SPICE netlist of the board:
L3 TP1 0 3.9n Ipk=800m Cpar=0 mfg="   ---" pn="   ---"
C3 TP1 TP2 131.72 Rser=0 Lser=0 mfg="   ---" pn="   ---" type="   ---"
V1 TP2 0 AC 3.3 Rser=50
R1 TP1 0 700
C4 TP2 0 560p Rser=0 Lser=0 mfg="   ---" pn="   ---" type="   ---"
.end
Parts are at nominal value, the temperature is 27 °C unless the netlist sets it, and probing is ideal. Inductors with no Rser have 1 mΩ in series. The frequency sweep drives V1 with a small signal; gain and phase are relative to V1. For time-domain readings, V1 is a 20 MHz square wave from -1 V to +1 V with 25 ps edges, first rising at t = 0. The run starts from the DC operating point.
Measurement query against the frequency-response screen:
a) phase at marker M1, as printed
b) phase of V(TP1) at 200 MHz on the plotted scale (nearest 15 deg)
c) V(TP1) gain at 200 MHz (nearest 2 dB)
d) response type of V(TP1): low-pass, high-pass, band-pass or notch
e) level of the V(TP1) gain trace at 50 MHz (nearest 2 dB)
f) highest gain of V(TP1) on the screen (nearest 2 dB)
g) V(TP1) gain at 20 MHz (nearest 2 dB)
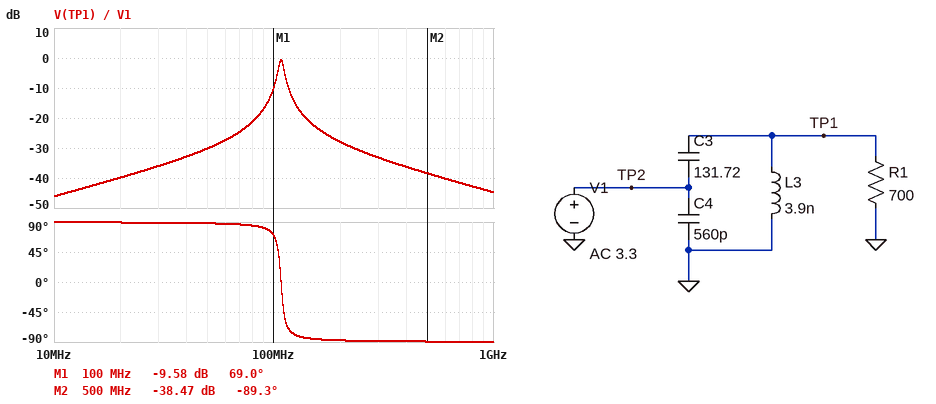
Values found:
69.0 deg
-90 deg
-28 dB
band-pass
-30 dB
0 dB
-40 dB
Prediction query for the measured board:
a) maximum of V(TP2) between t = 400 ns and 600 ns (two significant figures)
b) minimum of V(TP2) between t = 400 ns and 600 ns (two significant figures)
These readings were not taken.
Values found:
-890 mV
-1.1 V
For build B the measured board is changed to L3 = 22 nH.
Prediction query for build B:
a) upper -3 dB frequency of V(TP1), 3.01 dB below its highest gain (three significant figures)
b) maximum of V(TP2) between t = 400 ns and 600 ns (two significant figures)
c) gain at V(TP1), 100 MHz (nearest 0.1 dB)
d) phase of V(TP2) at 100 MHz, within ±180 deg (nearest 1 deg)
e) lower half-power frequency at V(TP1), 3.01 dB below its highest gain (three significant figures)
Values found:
48.5 MHz
-850 mV
-22.9 dB
-86 deg
42.4 MHz
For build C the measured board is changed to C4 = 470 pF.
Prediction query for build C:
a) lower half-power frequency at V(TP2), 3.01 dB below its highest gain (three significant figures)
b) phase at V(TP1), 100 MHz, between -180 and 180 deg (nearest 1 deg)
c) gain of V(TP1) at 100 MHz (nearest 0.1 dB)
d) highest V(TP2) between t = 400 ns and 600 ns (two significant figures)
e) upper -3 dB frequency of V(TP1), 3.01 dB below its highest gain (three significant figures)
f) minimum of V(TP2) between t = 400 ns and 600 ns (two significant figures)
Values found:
114 MHz
79 deg
-15.2 dB
-930 mV
121 MHz
-1.1 V
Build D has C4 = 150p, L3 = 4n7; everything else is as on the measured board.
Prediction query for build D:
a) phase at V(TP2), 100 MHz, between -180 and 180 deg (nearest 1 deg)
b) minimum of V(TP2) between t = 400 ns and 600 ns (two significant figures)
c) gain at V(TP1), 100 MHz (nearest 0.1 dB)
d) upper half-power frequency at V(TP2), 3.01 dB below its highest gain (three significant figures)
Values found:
85 deg
-1.2 V
-21.8 dB
201 MHz
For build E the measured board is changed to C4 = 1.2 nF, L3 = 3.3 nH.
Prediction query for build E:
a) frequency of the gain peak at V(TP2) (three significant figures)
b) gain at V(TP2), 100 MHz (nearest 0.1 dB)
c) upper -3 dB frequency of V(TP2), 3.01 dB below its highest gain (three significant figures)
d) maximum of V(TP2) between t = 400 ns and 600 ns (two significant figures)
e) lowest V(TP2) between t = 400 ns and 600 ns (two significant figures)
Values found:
80.0 MHz
-22.7 dB
81.4 MHz
-960 mV
-1.0 V
